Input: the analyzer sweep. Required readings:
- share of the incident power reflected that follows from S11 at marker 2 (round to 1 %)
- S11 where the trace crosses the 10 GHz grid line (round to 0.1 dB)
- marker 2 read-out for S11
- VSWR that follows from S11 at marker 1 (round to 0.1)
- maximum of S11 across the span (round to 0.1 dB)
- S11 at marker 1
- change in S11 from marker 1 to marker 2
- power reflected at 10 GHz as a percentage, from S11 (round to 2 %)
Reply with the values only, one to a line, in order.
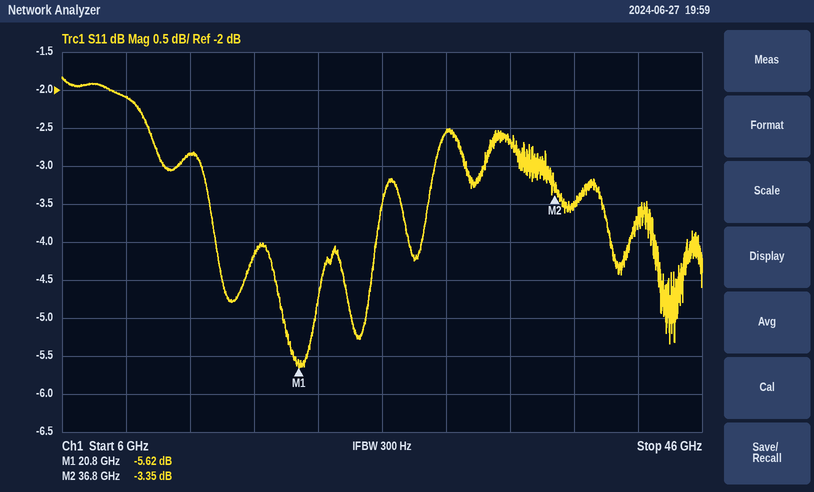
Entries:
46 %
-2.1 dB
-3.35 dB
3.2
-1.8 dB
-5.62 dB
2.27 dB
62 %
